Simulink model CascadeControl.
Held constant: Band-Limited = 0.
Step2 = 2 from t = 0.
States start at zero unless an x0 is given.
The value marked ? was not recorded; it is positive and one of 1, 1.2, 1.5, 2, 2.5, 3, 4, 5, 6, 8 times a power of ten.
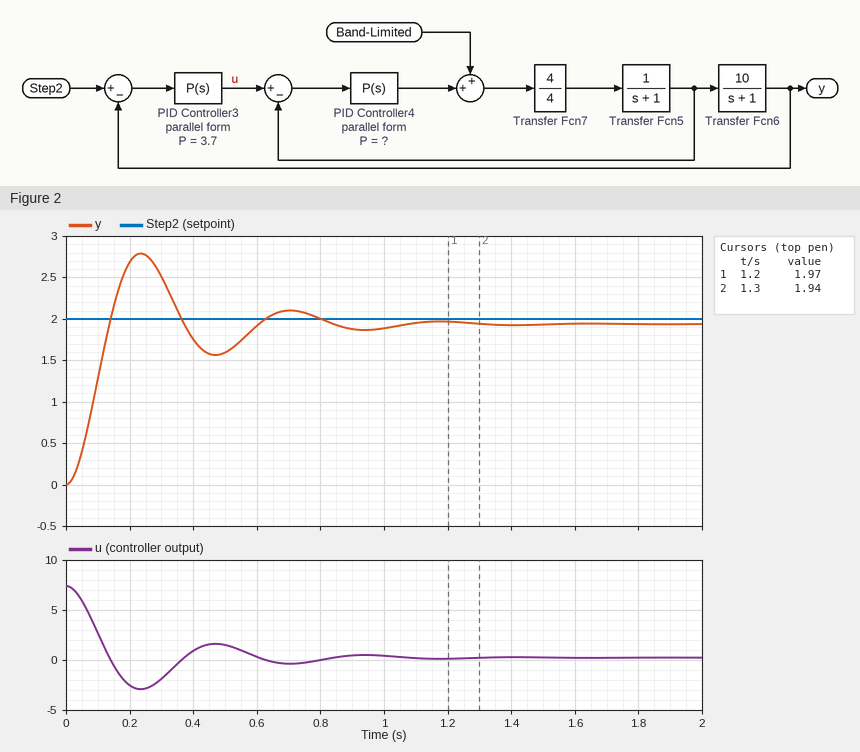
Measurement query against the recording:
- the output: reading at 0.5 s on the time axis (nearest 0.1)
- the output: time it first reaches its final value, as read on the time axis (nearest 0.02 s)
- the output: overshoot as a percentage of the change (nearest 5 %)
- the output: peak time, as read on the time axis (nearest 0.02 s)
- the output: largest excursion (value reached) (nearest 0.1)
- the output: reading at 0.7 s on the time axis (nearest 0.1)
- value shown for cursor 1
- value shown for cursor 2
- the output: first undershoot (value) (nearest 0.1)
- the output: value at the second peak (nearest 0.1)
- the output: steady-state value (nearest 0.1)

1.6
0.14 s
45 %
0.24 s
2.8
2.1
1.97
1.94
1.6
2.1
1.9
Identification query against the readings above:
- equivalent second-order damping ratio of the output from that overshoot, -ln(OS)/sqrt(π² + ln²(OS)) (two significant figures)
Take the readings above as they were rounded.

0.25
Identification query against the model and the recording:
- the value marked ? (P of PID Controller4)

5
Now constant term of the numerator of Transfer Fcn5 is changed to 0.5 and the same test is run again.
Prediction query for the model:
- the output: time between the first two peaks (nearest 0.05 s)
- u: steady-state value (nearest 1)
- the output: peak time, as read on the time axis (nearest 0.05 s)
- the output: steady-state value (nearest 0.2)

0.65 s
0
0.35 s
2.0
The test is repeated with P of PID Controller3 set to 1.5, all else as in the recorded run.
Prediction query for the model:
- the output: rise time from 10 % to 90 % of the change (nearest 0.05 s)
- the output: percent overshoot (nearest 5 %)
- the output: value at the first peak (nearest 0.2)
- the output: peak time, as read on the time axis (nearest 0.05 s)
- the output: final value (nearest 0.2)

0.15 s
25 %
2.4
0.40 s
1.8
